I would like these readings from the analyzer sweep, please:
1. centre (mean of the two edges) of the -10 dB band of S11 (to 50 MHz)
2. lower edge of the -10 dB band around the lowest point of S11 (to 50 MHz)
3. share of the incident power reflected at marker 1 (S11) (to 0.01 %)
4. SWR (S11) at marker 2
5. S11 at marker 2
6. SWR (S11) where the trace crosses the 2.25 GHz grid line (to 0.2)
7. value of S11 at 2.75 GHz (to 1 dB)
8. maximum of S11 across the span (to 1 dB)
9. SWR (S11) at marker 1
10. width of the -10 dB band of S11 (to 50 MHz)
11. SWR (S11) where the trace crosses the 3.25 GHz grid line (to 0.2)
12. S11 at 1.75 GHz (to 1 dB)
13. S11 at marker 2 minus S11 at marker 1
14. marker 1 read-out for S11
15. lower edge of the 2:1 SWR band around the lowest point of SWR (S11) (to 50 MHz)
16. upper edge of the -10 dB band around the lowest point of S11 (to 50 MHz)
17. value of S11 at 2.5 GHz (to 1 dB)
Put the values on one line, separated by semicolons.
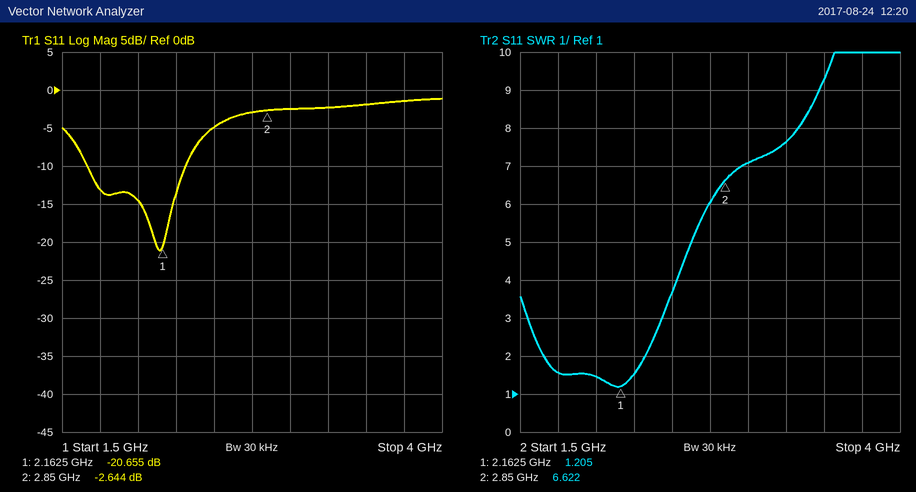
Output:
2.00 GHz; 1.65 GHz; 0.86 %; 6.622; -2.644 dB; 1.6; -3 dB; -1 dB; 1.205; 650 MHz; 7.6; -13 dB; 18.011 dB; -20.655 dB; 1.65 GHz; 2.30 GHz; -5 dB
